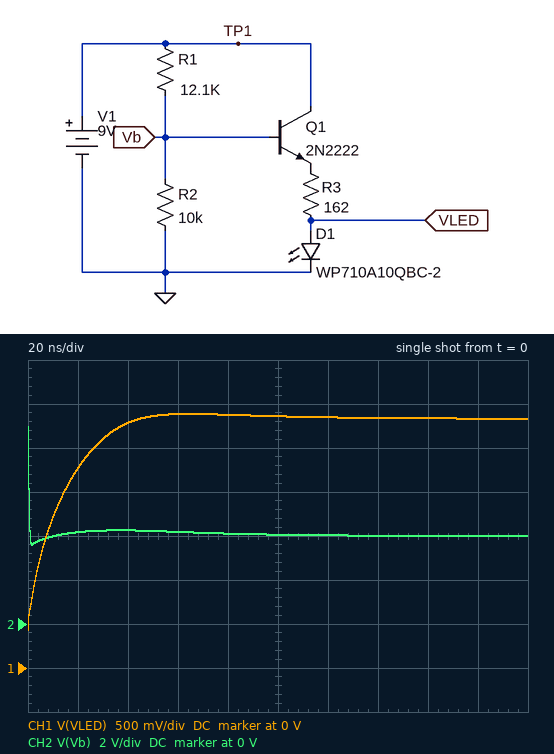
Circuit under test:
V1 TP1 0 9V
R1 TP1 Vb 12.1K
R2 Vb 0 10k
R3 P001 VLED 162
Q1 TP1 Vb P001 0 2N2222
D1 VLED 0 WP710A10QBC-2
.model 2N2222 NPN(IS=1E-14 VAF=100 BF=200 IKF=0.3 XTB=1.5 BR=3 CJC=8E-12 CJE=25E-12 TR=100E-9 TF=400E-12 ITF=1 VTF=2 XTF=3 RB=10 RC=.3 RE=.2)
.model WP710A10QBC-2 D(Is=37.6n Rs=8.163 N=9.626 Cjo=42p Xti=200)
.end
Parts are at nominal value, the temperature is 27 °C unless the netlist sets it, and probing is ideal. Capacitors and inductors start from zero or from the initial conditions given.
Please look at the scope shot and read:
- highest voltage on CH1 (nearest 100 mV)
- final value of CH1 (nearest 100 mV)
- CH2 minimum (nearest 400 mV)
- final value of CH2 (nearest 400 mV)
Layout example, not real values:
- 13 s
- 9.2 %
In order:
- 2.9 V
- 2.8 V
- 3.6 V
- 4.0 V
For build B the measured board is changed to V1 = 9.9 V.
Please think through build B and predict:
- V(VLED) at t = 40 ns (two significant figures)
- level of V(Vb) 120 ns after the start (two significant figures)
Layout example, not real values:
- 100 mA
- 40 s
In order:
- 3.0 V
- 4.4 V
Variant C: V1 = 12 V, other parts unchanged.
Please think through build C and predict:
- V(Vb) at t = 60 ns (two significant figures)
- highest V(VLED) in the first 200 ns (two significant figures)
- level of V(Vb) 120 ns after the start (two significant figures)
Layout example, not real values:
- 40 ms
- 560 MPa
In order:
- 5.4 V
- 3.2 V
- 5.2 V
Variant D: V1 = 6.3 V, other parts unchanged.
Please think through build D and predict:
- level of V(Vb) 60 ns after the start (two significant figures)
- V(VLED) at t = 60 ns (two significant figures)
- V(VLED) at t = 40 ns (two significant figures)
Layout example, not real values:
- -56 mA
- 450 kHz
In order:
- 2.9 V
- 2.0 V
- 1.7 V
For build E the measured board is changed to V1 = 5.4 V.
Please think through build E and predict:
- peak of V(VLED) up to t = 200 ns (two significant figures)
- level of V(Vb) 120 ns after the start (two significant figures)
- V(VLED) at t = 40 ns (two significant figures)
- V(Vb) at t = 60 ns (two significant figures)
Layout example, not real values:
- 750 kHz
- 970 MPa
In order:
- 1.9 V
- 2.5 V
- 1.3 V
- 2.4 V
